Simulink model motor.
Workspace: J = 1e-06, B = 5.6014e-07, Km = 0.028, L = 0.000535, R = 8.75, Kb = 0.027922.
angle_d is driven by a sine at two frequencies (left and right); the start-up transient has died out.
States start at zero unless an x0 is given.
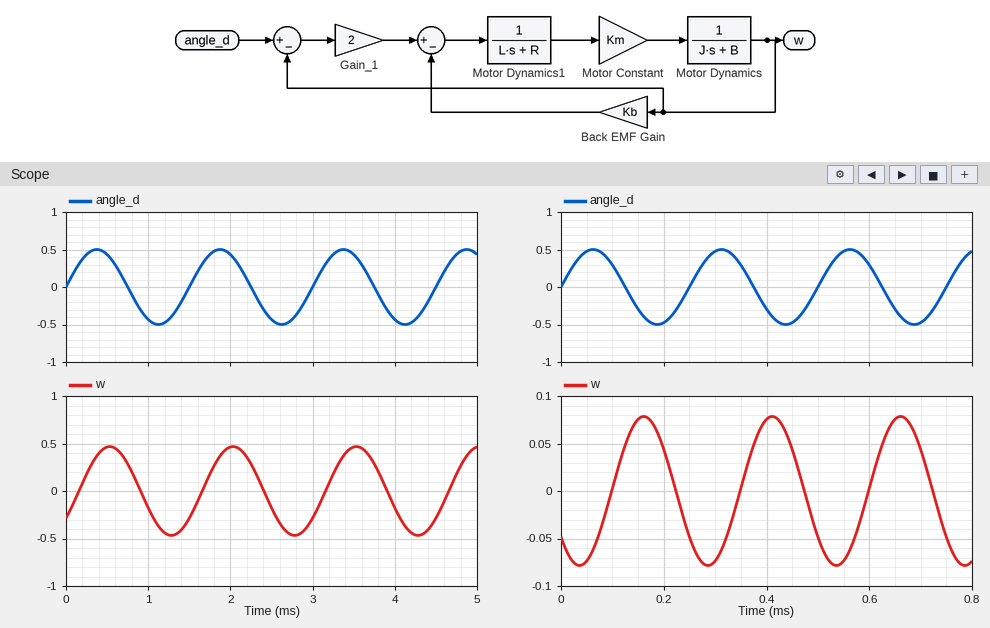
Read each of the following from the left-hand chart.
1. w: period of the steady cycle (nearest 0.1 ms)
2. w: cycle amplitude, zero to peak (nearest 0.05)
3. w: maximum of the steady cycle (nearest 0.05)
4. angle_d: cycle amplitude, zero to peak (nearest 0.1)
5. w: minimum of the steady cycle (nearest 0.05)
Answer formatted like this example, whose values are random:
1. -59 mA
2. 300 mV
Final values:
1. 1.5 ms
2. 0.45
3. 0.45
4. 0.5
5. -0.45
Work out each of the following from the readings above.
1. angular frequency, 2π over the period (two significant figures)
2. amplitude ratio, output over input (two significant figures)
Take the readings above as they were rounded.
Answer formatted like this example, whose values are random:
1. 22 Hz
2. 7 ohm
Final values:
1. 4.2 rad/ms
2. 0.90
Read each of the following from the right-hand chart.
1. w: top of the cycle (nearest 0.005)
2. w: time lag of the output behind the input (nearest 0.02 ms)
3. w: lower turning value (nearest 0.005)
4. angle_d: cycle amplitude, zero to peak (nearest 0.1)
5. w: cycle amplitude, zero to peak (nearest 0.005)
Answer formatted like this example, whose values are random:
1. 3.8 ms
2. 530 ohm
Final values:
1. 0.080
2. 0.10 ms
3. -0.080
4. 0.5
5. 0.080
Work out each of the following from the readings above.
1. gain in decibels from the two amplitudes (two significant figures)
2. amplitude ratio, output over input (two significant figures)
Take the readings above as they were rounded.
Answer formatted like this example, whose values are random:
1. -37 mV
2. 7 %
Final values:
1. -16 dB
2. 0.16
